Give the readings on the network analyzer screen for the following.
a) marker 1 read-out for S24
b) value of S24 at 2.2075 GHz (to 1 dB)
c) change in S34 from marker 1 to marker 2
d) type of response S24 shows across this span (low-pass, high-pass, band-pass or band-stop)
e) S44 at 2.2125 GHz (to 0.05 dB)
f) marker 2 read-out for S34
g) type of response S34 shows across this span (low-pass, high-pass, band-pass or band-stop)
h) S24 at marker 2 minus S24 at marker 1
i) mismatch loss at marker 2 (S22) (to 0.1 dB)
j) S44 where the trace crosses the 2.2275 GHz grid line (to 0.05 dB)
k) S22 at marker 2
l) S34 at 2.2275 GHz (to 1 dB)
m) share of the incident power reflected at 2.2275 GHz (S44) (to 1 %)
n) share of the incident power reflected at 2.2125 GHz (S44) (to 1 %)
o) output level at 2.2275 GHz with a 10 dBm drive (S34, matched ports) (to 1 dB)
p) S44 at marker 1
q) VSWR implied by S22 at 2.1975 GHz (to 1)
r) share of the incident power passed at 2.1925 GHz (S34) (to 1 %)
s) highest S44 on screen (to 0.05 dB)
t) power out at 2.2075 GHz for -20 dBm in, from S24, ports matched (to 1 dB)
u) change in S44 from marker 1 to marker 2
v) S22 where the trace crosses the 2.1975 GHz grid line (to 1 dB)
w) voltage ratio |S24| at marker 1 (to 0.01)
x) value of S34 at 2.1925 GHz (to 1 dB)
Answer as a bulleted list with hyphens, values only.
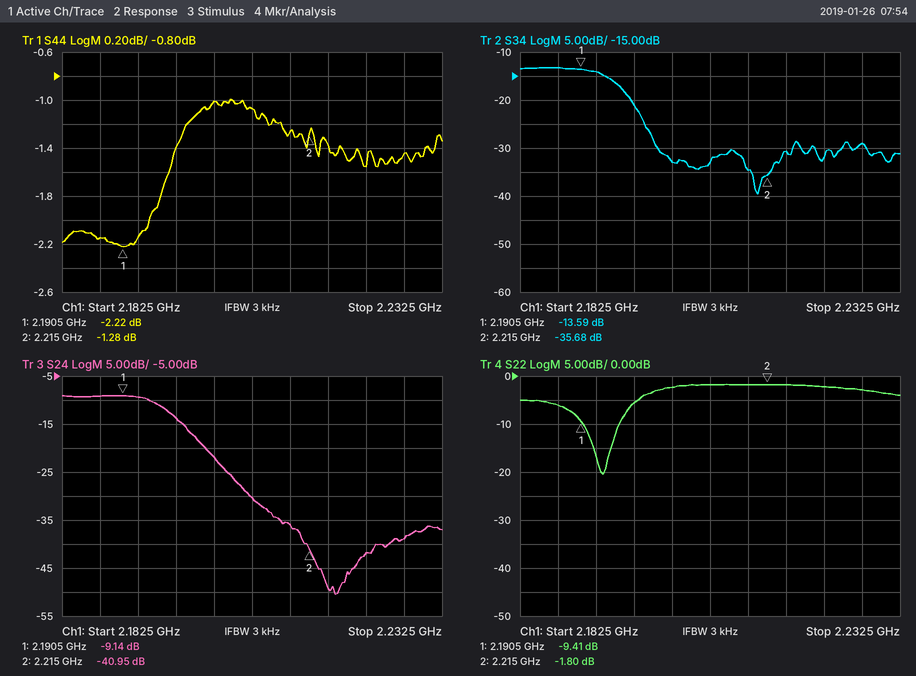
- -9.14 dB
- -30 dB
- -22.09 dB
- low-pass
- -1.25 dB
- -35.68 dB
- low-pass
- -31.81 dB
- 4.7 dB
- -1.45 dB
- -1.80 dB
- -29 dB
- 72 %
- 75 %
- -19 dBm
- -2.22 dB
- 3
- 4 %
- -1.00 dB
- -50 dBm
- 0.94 dB
- -6 dB
- 0.35
- -14 dB
